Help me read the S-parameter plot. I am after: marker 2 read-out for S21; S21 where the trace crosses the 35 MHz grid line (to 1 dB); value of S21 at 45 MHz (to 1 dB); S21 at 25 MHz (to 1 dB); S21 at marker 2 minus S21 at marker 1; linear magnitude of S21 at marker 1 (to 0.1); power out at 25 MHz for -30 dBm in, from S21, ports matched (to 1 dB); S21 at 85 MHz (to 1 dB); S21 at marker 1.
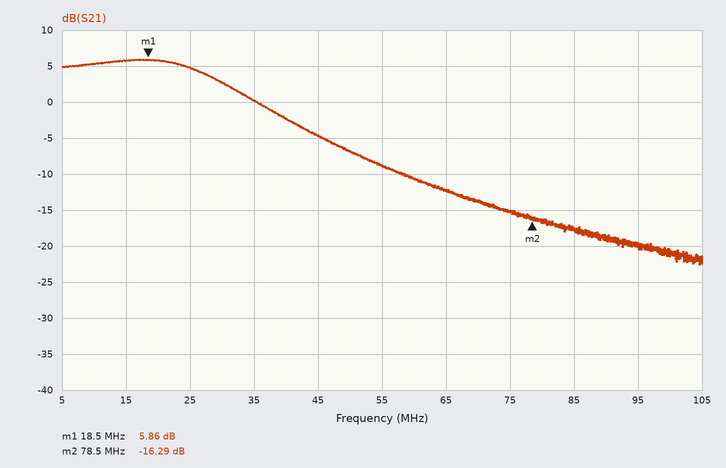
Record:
-16.29 dB
0 dB
-5 dB
5 dB
-22.15 dB
2.0
-25 dBm
-18 dB
5.86 dB
